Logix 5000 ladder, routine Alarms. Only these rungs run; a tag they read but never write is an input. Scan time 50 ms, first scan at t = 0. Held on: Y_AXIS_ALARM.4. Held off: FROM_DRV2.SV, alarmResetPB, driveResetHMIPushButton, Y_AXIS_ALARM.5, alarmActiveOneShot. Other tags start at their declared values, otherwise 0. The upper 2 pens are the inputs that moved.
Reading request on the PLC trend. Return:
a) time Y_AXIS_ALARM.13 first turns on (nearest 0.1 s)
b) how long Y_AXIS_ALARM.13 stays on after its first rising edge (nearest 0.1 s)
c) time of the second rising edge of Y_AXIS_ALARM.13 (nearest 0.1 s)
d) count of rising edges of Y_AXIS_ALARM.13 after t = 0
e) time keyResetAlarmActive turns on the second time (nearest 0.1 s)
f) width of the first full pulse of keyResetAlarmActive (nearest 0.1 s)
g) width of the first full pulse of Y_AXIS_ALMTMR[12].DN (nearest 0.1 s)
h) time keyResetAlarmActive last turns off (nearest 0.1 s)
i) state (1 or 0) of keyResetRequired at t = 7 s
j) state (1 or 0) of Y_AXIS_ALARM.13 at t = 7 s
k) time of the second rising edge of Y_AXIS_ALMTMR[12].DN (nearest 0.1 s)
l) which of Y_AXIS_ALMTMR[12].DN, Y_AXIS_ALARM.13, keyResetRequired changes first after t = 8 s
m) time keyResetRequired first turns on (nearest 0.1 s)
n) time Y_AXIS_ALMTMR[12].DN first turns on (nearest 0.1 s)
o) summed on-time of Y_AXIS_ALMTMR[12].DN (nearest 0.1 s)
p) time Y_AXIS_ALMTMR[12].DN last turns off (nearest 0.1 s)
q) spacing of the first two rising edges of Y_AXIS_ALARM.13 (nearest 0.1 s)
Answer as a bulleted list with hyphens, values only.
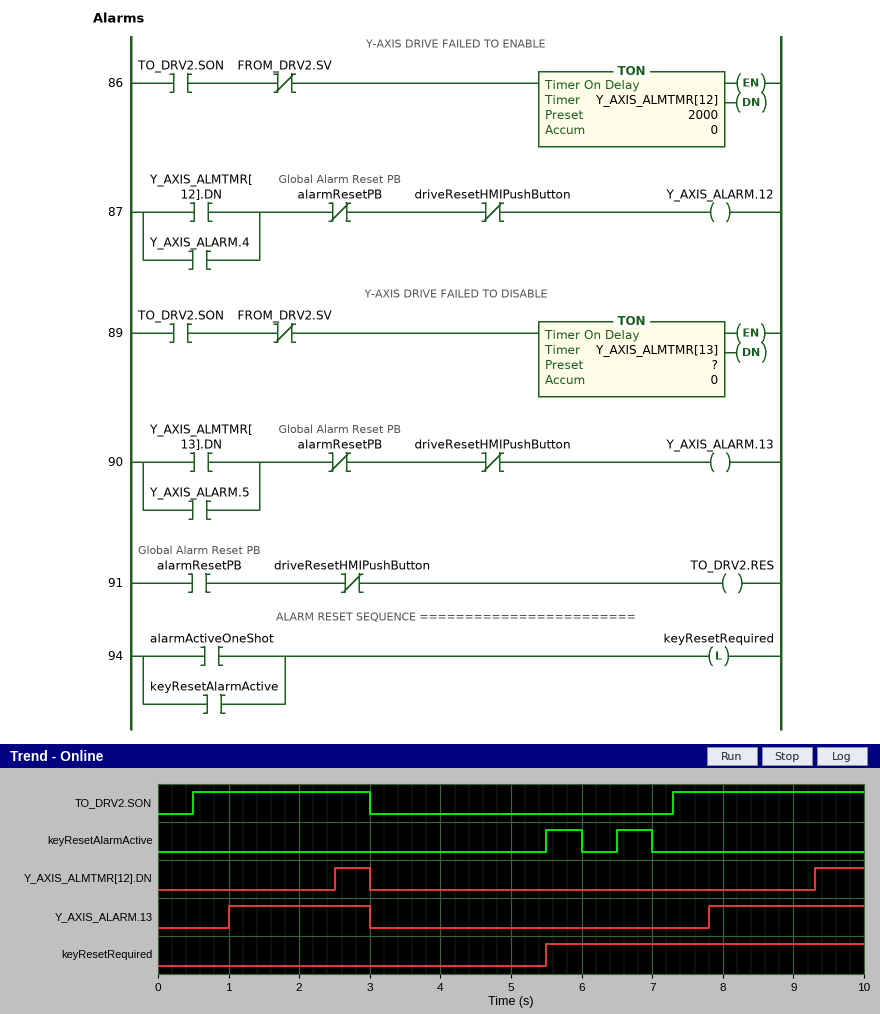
- 1.0 s
- 2.0 s
- 7.8 s
- 2
- 6.5 s
- 0.5 s
- 0.5 s
- 7.0 s
- 1
- 0
- 9.3 s
- Y_AXIS_ALMTMR[12].DN
- 5.5 s
- 2.5 s
- 1.2 s
- 3.0 s
- 6.8 s
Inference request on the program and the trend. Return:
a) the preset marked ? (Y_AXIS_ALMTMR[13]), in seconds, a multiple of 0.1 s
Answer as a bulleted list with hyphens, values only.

- 0.5 s
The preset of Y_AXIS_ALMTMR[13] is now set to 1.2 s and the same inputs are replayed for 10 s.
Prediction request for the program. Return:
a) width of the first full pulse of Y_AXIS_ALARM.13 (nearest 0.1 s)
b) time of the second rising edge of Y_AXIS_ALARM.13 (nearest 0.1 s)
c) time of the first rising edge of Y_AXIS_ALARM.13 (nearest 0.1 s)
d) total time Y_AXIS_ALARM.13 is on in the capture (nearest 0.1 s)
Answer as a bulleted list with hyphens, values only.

- 1.3 s
- 8.5 s
- 1.7 s
- 2.8 s
